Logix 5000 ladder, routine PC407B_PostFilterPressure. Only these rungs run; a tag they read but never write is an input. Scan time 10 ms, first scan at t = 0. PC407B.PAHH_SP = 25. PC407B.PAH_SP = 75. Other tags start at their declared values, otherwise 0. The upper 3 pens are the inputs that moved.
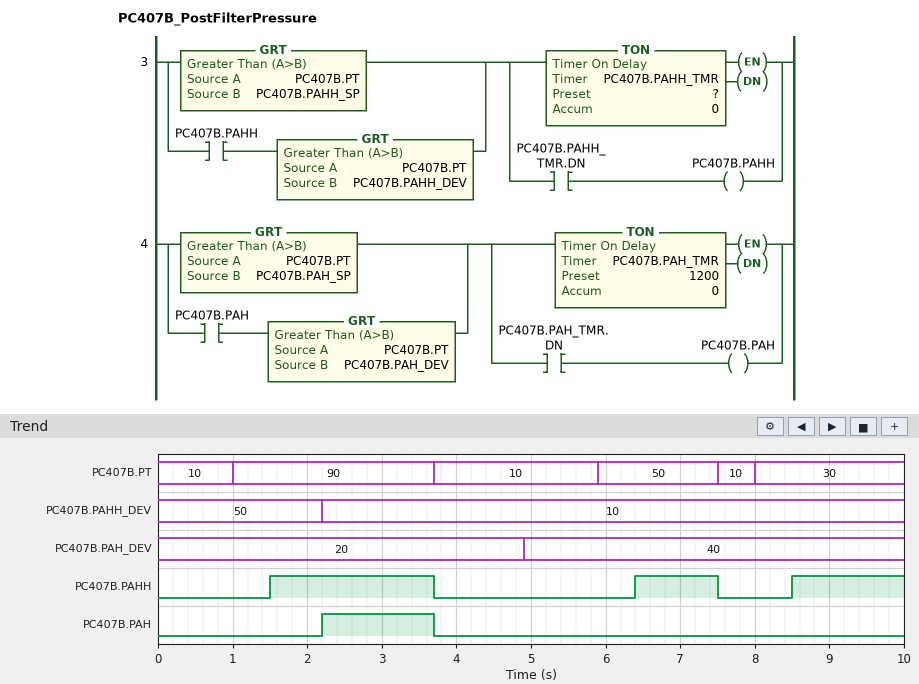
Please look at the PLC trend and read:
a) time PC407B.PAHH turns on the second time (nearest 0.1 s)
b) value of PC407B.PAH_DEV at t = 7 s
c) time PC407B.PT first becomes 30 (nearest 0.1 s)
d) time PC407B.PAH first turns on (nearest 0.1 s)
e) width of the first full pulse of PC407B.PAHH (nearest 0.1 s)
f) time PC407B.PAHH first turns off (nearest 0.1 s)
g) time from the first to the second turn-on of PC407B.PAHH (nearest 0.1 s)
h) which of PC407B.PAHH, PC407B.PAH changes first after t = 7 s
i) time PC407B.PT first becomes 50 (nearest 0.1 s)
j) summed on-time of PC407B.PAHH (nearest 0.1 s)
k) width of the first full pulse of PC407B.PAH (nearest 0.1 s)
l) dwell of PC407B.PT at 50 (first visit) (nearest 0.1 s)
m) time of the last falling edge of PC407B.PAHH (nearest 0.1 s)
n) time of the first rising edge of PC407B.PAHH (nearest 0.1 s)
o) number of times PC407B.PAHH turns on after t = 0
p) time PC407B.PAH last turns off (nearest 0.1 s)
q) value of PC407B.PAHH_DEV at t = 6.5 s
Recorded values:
6.4 s
40
8.0 s
2.2 s
2.2 s
3.7 s
4.9 s
PC407B.PAHH
5.9 s
4.8 s
1.5 s
1.6 s
7.5 s
1.5 s
3
3.7 s
10
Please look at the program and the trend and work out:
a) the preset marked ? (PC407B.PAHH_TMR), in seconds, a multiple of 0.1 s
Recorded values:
0.5 s
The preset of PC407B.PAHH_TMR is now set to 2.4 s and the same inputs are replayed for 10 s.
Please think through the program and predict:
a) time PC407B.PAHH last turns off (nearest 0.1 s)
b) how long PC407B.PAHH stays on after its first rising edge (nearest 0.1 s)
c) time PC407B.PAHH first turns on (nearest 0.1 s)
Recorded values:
3.7 s
0.3 s
3.4 s
